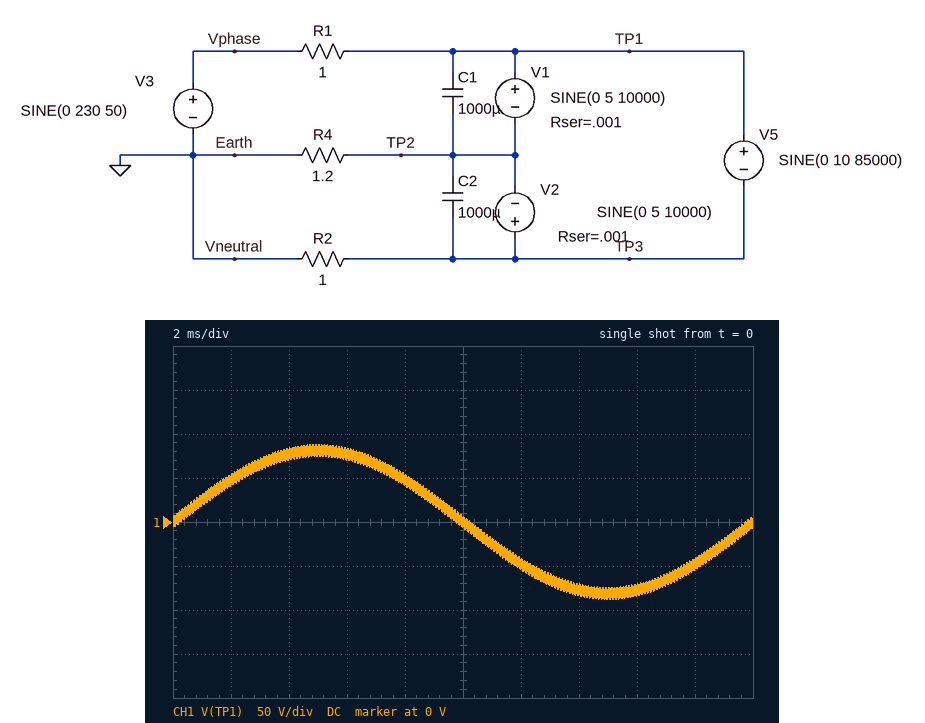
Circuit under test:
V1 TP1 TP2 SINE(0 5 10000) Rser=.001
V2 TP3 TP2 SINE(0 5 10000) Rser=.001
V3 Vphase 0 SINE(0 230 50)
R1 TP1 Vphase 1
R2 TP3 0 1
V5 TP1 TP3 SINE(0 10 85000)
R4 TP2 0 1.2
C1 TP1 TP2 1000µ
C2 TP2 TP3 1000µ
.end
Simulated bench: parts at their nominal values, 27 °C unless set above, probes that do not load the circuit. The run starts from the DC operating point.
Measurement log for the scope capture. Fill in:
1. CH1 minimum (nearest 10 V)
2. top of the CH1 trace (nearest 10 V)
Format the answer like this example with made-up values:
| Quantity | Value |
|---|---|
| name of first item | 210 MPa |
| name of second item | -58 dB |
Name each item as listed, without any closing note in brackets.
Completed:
| Quantity | Value |
|---|---|
| CH1 minimum | -90 V |
| top of the CH1 trace | 90 V |
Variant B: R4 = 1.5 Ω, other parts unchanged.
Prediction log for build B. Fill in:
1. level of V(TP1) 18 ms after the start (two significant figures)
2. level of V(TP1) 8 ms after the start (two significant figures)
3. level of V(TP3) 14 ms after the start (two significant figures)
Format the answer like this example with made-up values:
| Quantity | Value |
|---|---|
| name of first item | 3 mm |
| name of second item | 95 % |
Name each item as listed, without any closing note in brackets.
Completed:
| Quantity | Value |
|---|---|
| level of V(TP1) 18 ms after the start | -51 V |
| level of V(TP1) 8 ms after the start | 51 V |
| level of V(TP3) 14 ms after the start | -82 V |
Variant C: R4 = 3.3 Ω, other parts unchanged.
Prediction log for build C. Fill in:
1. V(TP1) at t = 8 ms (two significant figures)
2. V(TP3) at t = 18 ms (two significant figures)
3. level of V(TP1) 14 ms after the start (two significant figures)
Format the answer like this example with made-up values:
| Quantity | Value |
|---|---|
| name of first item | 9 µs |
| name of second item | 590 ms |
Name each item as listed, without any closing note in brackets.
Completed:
| Quantity | Value |
|---|---|
| V(TP1) at t = 8 ms | 59 V |
| V(TP3) at t = 18 ms | -59 V |
| level of V(TP1) 14 ms after the start | -95 V |
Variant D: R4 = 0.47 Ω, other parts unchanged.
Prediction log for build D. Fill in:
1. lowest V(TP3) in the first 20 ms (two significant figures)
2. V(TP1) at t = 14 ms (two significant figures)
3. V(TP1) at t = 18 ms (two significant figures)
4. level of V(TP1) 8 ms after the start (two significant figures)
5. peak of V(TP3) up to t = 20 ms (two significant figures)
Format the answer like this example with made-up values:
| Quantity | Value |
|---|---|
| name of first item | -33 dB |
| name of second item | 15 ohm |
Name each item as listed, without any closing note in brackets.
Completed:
| Quantity | Value |
|---|---|
| lowest V(TP3) in the first 20 ms | -63 V |
| V(TP1) at t = 14 ms | -53 V |
| V(TP1) at t = 18 ms | -33 V |
| level of V(TP1) 8 ms after the start | 33 V |
| peak of V(TP3) up to t = 20 ms | 63 V |
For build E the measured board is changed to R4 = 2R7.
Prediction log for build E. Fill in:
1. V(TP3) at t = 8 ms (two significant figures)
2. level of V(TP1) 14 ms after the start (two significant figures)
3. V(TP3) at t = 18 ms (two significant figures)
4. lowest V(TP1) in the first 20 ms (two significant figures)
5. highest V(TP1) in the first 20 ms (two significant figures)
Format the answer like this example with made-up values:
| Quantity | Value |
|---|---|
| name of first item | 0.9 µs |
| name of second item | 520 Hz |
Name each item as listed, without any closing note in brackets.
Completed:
| Quantity | Value |
|---|---|
| V(TP3) at t = 8 ms | 57 V |
| level of V(TP1) 14 ms after the start | -92 V |
| V(TP3) at t = 18 ms | -57 V |
| lowest V(TP1) in the first 20 ms | -100 V |
| highest V(TP1) in the first 20 ms | 100 V |
